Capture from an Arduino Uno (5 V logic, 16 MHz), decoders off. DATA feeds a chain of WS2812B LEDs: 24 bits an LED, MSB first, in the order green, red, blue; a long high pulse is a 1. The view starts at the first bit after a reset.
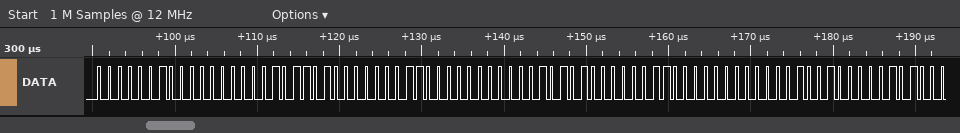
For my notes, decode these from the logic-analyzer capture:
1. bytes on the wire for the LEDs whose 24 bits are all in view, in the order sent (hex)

02 00 5A 03 00 15 03 00 09
